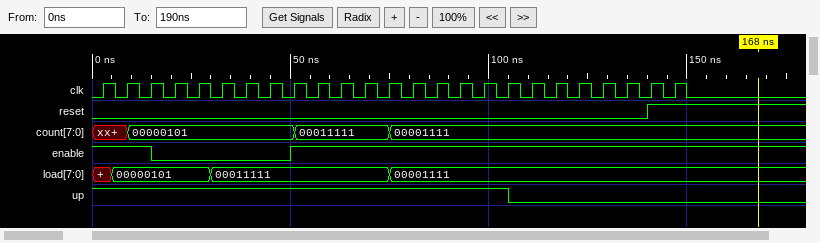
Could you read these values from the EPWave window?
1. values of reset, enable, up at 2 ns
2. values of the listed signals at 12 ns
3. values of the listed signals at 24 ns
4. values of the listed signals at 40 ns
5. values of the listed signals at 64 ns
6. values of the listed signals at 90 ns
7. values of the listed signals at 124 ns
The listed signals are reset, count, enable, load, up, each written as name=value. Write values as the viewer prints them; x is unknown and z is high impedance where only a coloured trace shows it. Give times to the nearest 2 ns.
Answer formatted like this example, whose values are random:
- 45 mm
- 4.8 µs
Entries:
- reset=0, enable=1, up=1
- reset=0, count=00000101, enable=1, load=00000101, up=1
- reset=0, count=00000101, enable=0, load=00000101, up=1
- reset=0, count=00000101, enable=0, load=00011111, up=1
- reset=0, count=00011111, enable=1, load=00011111, up=1
- reset=0, count=00001111, enable=1, load=00001111, up=1
- reset=0, count=00001111, enable=1, load=00001111, up=0
